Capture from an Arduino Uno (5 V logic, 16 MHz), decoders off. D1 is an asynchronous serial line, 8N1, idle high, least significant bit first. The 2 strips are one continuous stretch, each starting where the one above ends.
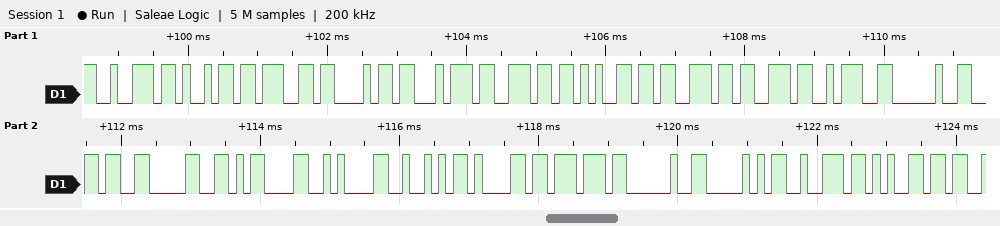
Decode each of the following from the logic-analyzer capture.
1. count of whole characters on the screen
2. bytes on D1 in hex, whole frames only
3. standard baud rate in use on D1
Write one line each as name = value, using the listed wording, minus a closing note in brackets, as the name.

count of whole characters on the screen = 22
bytes on D1 in hex, whole frames only = 72 69 67 68 74 6E 65 73 73 3A 20 36 30 0D 0A 52 61 77 20 50 72 65
standard baud rate in use on D1 = 9600 baud
